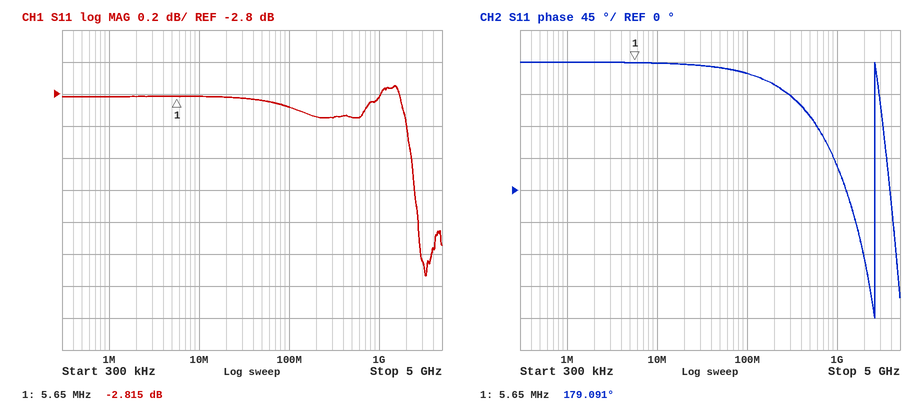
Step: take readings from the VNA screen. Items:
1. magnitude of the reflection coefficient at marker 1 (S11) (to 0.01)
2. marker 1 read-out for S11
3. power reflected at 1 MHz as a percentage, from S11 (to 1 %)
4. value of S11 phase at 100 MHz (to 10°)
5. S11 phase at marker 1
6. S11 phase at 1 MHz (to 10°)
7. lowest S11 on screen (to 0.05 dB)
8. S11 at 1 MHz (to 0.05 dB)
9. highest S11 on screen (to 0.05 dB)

0.72
-2.815 dB
52 %
160°
179.091°
180°
-3.95 dB
-2.80 dB
-2.75 dB
